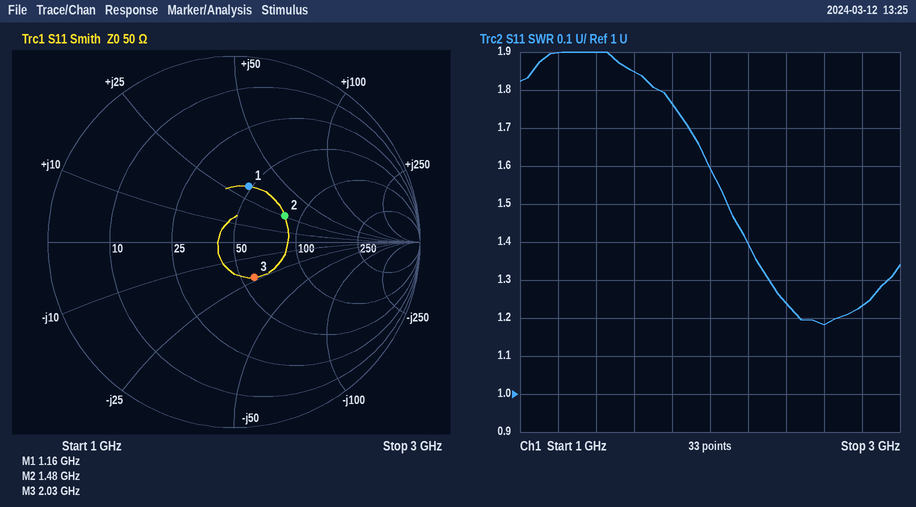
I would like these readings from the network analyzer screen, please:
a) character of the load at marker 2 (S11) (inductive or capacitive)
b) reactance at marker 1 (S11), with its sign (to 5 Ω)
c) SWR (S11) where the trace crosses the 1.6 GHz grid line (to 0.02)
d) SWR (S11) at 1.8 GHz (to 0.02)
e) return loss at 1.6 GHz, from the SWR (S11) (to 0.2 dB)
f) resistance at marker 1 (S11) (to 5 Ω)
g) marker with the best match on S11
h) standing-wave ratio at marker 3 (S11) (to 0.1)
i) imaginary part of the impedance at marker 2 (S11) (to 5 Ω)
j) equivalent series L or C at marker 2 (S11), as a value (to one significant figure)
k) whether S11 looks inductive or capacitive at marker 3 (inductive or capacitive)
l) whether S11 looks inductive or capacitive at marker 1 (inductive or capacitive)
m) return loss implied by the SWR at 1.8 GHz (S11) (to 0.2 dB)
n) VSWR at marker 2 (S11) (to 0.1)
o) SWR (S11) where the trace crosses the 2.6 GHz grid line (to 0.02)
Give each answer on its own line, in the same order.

inductive
+30 Ω
1.84
1.76
10.6 dB
50 Ω
marker 3
1.6
+25 Ω
3 nH
capacitive
inductive
11.2 dB
1.9
1.18
